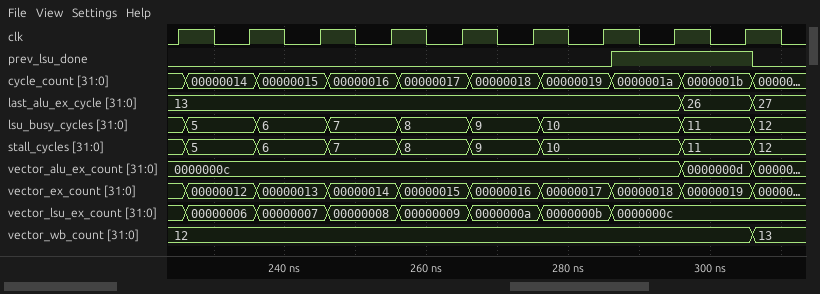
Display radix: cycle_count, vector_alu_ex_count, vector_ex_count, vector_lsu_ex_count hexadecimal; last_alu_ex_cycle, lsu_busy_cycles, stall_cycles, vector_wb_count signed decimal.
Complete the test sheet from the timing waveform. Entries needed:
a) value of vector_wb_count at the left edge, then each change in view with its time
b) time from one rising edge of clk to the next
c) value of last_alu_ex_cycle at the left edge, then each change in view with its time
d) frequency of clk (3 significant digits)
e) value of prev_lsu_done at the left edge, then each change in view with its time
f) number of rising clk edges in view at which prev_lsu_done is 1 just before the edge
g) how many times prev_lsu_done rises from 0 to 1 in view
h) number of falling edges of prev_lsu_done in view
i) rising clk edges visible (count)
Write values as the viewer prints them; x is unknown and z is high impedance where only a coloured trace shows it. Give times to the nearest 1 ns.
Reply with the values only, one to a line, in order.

12, 13 at 306 ns
10 ns
13, 26 at 296 ns, 27 at 306 ns
100 MHz
0, 1 at 286 ns, 0 at 306 ns
2
1
1
9
